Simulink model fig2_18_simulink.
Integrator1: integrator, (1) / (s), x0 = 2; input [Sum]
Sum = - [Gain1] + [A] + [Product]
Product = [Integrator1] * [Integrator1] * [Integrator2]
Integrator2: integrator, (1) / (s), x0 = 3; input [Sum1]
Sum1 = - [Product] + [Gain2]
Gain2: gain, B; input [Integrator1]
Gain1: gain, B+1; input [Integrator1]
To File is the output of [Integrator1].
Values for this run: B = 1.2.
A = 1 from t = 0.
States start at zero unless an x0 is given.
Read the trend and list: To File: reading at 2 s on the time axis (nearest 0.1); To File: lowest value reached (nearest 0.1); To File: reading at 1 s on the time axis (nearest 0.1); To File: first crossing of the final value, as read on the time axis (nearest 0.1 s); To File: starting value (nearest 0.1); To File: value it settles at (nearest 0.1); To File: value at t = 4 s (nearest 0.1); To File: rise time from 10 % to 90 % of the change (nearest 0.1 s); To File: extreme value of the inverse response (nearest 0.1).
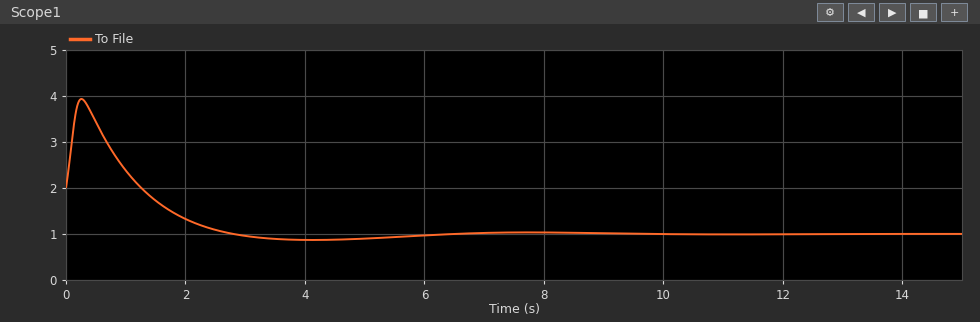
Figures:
1.3
0.9
2.4
2.8 s
2.0
1.0
0.9
1.1 s
3.9
